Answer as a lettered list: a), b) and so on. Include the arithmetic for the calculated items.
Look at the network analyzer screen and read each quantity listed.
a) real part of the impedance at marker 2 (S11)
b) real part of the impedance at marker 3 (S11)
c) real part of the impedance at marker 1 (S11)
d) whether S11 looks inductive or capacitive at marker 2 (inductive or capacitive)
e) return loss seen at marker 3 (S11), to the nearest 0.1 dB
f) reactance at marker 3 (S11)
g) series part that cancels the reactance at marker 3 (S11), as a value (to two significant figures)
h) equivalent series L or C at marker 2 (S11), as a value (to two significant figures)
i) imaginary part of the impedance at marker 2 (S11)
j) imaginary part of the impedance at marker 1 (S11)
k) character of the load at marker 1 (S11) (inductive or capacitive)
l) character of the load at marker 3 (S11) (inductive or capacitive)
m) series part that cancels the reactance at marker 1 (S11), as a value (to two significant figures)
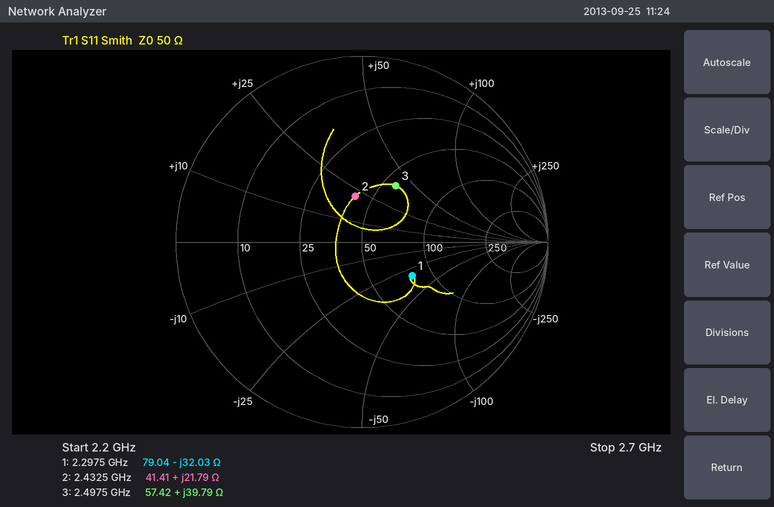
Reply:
a) 41.41 Ω
b) 57.42 Ω
c) 79.04 Ω
d) inductive
e) 9.0 dB
f) +39.79 Ω
g) C = 1/(2π × 2.4975 GHz × 39.79 Ω) ≈ 1.6 pF
h) L = 21.79 Ω/(2π × 2.4325 GHz) ≈ 1.4 nH
i) +21.79 Ω
j) -32.03 Ω
k) capacitive
l) inductive
m) L = 32.03 Ω/(2π × 2.2975 GHz) ≈ 2.2 nH
